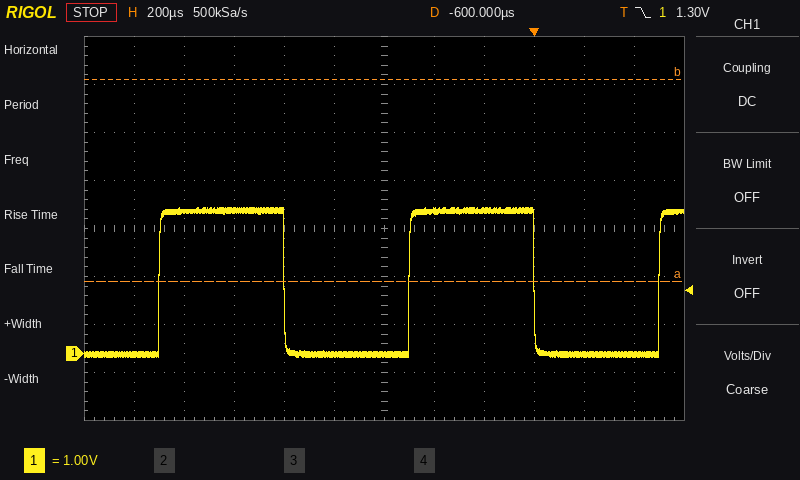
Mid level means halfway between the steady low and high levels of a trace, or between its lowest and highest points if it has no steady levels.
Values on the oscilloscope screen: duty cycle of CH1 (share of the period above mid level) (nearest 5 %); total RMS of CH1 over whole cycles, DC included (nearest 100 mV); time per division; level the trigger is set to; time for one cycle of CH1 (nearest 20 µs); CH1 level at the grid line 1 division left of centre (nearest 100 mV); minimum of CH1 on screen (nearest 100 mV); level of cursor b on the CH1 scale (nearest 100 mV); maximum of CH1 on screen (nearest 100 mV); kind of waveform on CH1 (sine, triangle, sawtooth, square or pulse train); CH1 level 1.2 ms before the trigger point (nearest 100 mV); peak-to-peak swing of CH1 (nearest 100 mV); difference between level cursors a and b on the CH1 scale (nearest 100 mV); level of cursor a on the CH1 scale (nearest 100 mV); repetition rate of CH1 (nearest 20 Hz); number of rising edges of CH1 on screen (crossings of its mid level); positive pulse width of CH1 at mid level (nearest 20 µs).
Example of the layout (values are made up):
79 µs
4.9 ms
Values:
50 %
2.1 V
200 µs
1.30 V
1.00 ms
0.0 V
-100 mV
5.7 V
3.0 V
square
3.0 V
3.1 V
4.2 V
1.5 V
1.00 kHz
3
500 µs
